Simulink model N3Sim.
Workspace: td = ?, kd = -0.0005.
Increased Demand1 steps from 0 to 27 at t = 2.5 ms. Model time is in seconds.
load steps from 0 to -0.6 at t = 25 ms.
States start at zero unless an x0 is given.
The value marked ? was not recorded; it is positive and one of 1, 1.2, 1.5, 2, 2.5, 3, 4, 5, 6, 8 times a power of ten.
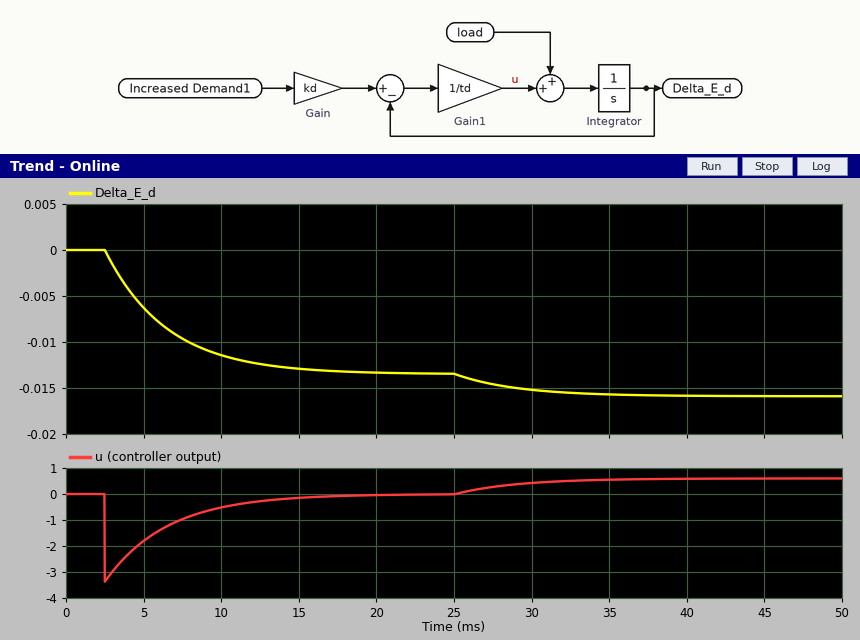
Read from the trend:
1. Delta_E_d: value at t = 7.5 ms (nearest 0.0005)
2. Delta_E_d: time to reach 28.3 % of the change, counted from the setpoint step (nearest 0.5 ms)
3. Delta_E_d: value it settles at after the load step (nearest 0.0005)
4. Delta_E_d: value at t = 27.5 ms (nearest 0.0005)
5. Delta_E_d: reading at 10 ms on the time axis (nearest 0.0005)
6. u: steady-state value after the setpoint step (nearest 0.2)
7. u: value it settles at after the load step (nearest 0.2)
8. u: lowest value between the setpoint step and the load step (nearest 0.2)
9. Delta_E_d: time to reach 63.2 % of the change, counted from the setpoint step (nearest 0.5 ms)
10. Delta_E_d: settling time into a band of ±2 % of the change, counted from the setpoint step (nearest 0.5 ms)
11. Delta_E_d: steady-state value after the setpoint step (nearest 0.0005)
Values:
-0.0095
1.5 ms
-0.0160
-0.0145
-0.0115
0.0
0.6
-3.4
4.0 ms
15.5 ms
-0.0135
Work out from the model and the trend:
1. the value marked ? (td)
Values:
0.004
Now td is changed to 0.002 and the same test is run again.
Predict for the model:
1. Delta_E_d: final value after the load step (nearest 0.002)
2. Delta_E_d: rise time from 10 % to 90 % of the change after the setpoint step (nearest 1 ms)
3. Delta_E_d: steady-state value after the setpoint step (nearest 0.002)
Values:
-0.014
4 ms
-0.014
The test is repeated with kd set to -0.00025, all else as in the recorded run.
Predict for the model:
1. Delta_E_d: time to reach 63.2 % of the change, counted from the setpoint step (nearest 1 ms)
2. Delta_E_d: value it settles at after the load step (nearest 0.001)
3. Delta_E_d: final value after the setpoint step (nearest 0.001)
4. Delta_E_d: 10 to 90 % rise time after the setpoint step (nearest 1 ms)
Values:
4 ms
-0.009
-0.007
9 ms
